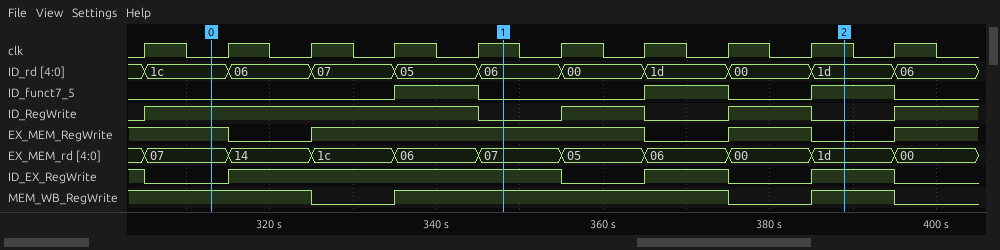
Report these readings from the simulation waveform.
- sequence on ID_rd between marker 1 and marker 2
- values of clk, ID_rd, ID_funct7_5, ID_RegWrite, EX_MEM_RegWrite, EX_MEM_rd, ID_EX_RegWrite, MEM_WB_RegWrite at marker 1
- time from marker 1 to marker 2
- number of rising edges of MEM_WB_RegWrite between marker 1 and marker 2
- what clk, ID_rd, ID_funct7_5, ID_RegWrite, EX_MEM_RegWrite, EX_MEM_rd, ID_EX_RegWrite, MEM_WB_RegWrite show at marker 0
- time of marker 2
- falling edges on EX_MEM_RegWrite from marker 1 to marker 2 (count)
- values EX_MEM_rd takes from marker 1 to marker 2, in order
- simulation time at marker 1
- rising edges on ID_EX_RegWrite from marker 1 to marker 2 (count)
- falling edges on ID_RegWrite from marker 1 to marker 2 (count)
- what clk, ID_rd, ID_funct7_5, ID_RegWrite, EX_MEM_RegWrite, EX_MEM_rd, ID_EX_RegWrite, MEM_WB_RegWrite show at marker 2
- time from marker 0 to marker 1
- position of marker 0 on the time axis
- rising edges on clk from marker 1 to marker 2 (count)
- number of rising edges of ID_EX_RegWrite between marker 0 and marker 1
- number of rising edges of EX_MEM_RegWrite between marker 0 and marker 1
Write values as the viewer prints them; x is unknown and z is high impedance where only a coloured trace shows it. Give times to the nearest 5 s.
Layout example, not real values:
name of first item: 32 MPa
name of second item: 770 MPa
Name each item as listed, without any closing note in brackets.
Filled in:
sequence on ID_rd between marker 1 and marker 2: 06, 00, 1d, 00, 1d
values of clk, ID_rd, ID_funct7_5, ID_RegWrite, EX_MEM_RegWrite, EX_MEM_rd, ID_EX_RegWrite, MEM_WB_RegWrite at marker 1: clk=1, ID_rd=06, ID_funct7_5=0, ID_RegWrite=0, EX_MEM_RegWrite=1, EX_MEM_rd=07, ID_EX_RegWrite=1, MEM_WB_RegWrite=1
time from marker 1 to marker 2: 40 s
number of rising edges of MEM_WB_RegWrite between marker 1 and marker 2: 1
what clk, ID_rd, ID_funct7_5, ID_RegWrite, EX_MEM_RegWrite, EX_MEM_rd, ID_EX_RegWrite, MEM_WB_RegWrite show at marker 0: clk=0, ID_rd=1c, ID_funct7_5=0, ID_RegWrite=1, EX_MEM_RegWrite=1, EX_MEM_rd=07, ID_EX_RegWrite=0, MEM_WB_RegWrite=1
time of marker 2: 390 s
falling edges on EX_MEM_RegWrite from marker 1 to marker 2: 2
values EX_MEM_rd takes from marker 1 to marker 2, in order: 07, 05, 06, 00, 1d
simulation time at marker 1: 350 s
rising edges on ID_EX_RegWrite from marker 1 to marker 2: 2
falling edges on ID_RegWrite from marker 1 to marker 2: 2
what clk, ID_rd, ID_funct7_5, ID_RegWrite, EX_MEM_RegWrite, EX_MEM_rd, ID_EX_RegWrite, MEM_WB_RegWrite show at marker 2: clk=1, ID_rd=1d, ID_funct7_5=1, ID_RegWrite=0, EX_MEM_RegWrite=0, EX_MEM_rd=1d, ID_EX_RegWrite=1, MEM_WB_RegWrite=1
time from marker 0 to marker 1: 35 s
position of marker 0 on the time axis: 315 s
rising edges on clk from marker 1 to marker 2: 4
number of rising edges of ID_EX_RegWrite between marker 0 and marker 1: 1
number of rising edges of EX_MEM_RegWrite between marker 0 and marker 1: 1
